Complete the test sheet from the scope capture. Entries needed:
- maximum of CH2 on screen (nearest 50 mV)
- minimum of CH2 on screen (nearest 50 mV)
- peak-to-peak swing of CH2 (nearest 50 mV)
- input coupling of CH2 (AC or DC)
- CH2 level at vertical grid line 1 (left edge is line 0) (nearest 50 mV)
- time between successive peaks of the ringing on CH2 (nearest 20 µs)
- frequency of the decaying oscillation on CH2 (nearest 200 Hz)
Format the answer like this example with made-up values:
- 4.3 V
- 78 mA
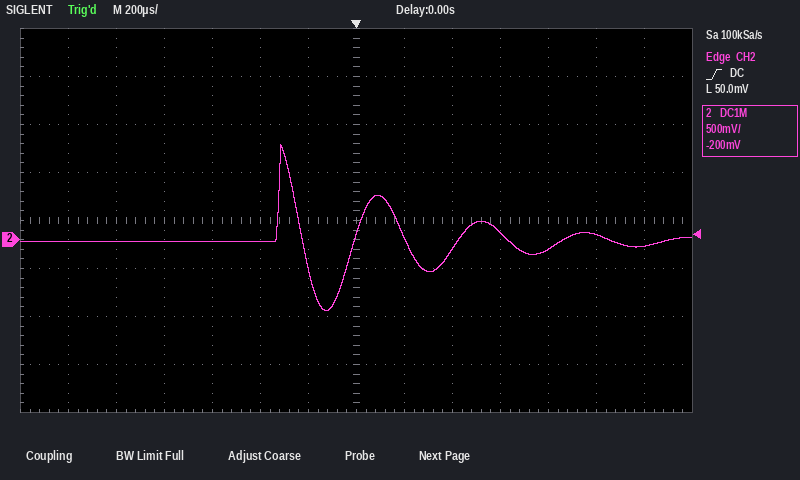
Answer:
- 1.00 V
- -750 mV
- 1.75 V
- DC
- 0 mV
- 420 µs
- 2.4 kHz
